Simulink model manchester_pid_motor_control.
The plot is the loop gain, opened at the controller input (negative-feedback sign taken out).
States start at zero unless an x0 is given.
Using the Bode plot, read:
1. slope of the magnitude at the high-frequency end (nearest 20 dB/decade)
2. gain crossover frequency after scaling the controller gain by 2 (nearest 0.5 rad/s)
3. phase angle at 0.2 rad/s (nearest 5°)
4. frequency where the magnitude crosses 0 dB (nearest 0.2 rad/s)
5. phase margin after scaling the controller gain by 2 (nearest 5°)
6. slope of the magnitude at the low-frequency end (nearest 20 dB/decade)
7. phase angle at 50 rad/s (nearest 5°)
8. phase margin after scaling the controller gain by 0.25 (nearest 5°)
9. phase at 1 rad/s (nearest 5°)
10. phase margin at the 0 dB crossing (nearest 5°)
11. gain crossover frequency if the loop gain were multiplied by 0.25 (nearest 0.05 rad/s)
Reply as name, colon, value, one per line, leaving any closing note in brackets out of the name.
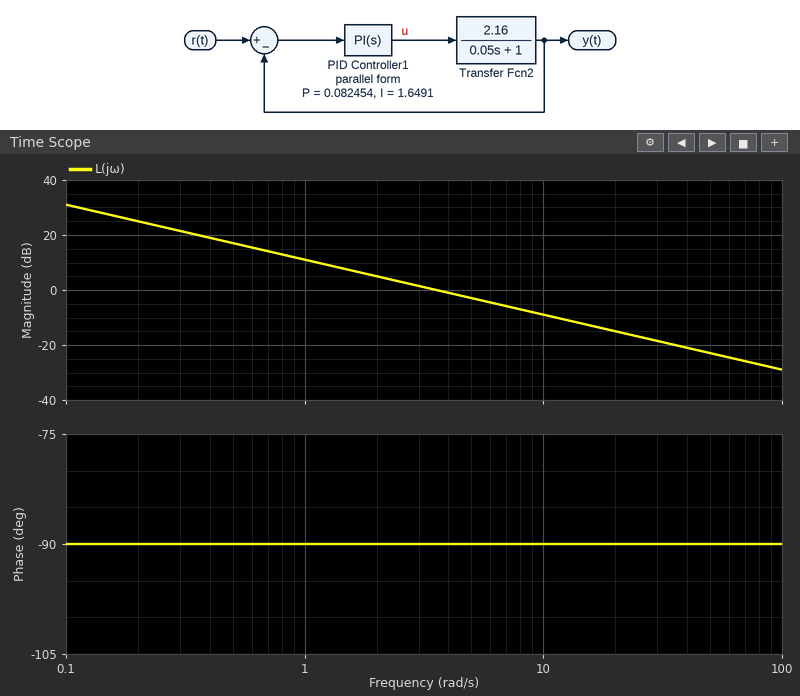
slope of the magnitude at the high-frequency end: -20 dB/decade
gain crossover frequency after scaling the controller gain by 2: 7.0 rad/s
phase angle at 0.2 rad/s: -90°
frequency where the magnitude crosses 0 dB: 3.6 rad/s
phase margin after scaling the controller gain by 2: 90°
slope of the magnitude at the low-frequency end: -20 dB/decade
phase angle at 50 rad/s: -90°
phase margin after scaling the controller gain by 0.25: 90°
phase at 1 rad/s: -90°
phase margin at the 0 dB crossing: 90°
gain crossover frequency if the loop gain were multiplied by 0.25: 0.90 rad/s
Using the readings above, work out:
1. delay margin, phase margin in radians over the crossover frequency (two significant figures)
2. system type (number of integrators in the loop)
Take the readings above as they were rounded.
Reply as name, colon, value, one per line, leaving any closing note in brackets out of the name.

delay margin, phase margin in radians over the crossover frequency: 0.44 s
system type: 1
